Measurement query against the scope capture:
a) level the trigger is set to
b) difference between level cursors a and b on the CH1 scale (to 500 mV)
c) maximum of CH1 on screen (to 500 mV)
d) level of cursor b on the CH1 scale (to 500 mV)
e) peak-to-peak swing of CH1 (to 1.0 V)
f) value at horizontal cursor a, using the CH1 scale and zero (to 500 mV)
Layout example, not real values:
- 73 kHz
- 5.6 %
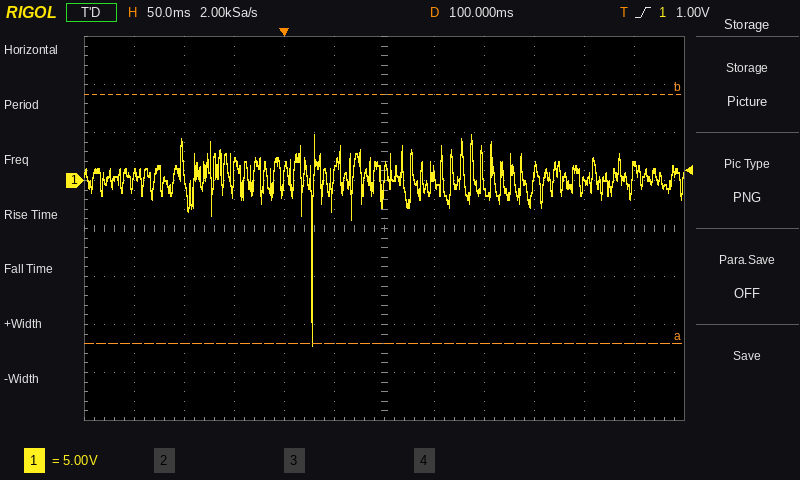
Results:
- 1.00 V
- 26.0 V
- 5.0 V
- 9.0 V
- 22.0 V
- -17.0 V
